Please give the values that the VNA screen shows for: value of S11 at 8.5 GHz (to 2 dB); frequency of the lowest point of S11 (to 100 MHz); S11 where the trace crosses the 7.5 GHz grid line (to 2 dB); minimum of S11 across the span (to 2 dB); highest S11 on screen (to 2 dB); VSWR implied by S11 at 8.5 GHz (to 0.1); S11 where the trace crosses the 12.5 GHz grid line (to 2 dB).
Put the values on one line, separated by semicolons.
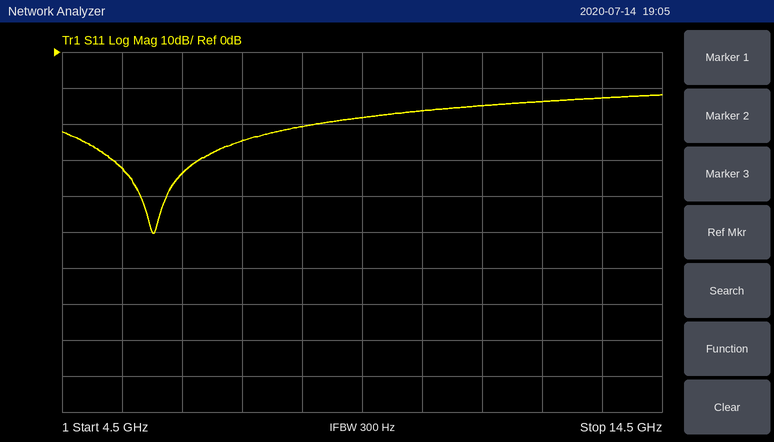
-20 dB; 6.0 GHz; -24 dB; -50 dB; -12 dB; 1.2; -14 dB
